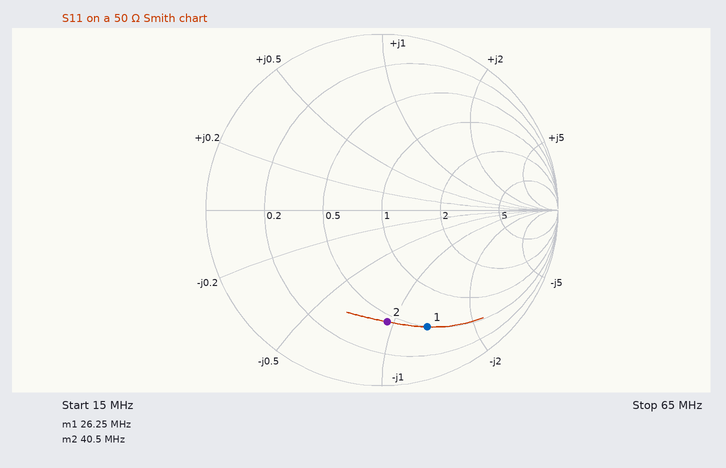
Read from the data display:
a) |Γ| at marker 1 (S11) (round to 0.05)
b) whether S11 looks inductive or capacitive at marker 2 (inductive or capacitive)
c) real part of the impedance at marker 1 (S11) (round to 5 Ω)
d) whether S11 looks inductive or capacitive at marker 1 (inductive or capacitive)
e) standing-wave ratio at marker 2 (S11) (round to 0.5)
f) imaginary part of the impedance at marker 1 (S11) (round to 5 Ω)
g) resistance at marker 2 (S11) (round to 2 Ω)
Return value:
0.70
capacitive
25 Ω
capacitive
4.5
-65 Ω
22 Ω
